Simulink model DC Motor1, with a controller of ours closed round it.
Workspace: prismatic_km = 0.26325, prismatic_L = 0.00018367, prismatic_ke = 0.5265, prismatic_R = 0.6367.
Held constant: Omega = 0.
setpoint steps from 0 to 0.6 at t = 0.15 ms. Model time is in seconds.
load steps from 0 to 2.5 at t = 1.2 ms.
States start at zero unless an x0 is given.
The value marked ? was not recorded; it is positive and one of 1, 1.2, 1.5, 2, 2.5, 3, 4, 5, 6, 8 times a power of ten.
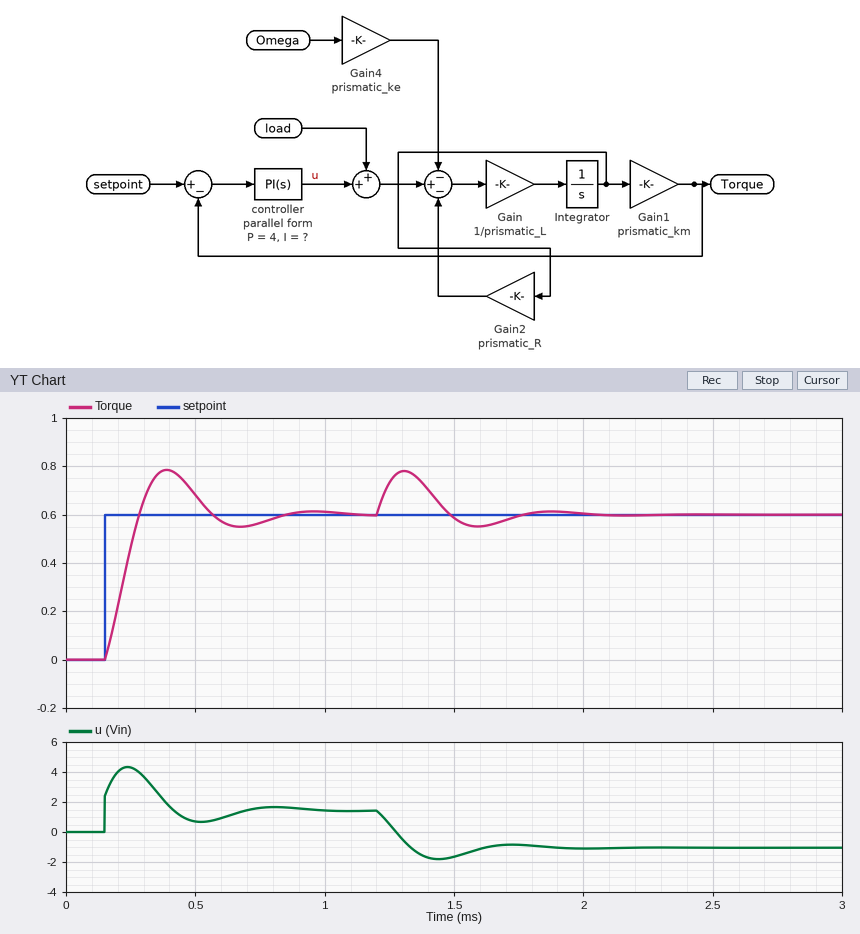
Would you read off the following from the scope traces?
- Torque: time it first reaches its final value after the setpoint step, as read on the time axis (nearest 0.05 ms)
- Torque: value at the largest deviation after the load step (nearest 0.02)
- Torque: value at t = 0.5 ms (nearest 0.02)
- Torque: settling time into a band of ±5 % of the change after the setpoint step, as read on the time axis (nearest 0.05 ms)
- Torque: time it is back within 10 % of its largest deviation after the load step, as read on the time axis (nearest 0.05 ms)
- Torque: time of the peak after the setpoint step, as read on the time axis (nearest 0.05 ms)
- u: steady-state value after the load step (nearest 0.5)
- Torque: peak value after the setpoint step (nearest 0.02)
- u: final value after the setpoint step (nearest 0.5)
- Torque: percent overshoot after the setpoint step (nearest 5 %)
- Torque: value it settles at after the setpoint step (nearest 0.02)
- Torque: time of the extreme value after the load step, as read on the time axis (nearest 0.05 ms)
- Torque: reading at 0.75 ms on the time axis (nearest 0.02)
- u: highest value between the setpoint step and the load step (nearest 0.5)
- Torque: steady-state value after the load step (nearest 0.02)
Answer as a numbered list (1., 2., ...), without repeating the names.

1. 0.30 ms
2. 0.78
3. 0.68
4. 0.75 ms
5. 1.70 ms
6. 0.40 ms
7. -1.0
8. 0.78
9. 1.5
10. 30 %
11. 0.60
12. 1.30 ms
13. 0.56
14. 4.5
15. 0.60
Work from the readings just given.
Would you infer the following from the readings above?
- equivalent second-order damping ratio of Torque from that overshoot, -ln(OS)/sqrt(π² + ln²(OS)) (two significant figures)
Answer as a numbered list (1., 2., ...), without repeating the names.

1. 0.36
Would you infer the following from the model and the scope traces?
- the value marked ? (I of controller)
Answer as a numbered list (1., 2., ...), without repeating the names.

1. 100000
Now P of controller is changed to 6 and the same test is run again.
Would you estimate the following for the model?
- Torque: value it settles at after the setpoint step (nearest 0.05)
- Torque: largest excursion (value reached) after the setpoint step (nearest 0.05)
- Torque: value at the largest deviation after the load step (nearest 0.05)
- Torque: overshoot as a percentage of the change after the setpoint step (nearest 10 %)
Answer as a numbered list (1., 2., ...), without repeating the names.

1. 0.60
2. 0.75
3. 0.75
4. 20 %
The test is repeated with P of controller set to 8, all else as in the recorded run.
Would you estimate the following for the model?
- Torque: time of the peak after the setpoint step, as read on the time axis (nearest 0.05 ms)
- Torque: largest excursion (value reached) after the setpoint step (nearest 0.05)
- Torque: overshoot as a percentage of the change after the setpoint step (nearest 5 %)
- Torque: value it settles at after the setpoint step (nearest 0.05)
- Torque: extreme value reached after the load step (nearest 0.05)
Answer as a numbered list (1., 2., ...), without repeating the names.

1. 0.35 ms
2. 0.70
3. 15 %
4. 0.60
5. 0.75
